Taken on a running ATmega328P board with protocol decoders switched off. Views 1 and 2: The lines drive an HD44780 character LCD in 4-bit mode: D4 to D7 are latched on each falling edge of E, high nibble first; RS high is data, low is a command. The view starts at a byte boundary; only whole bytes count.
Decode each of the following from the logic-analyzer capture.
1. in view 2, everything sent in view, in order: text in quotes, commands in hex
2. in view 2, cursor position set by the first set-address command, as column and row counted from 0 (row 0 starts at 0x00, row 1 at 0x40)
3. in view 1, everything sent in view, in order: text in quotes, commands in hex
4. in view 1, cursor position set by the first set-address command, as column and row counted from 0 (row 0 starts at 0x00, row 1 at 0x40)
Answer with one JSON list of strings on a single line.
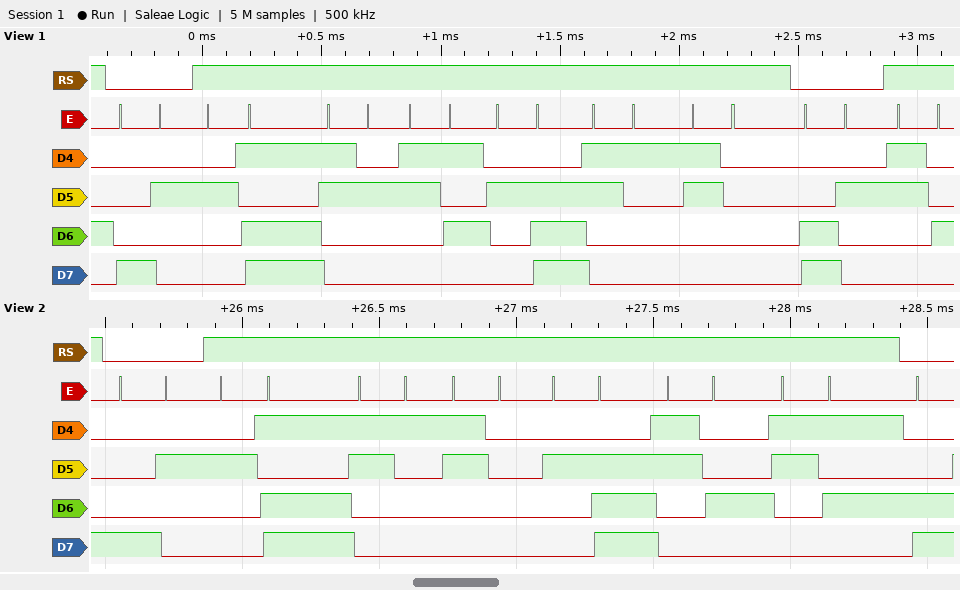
["0x82 \"-10.45\"", "column 2, row 0", "0x82 \"-25.10\" 0xC2 \"4\"", "column 2, row 0"]
